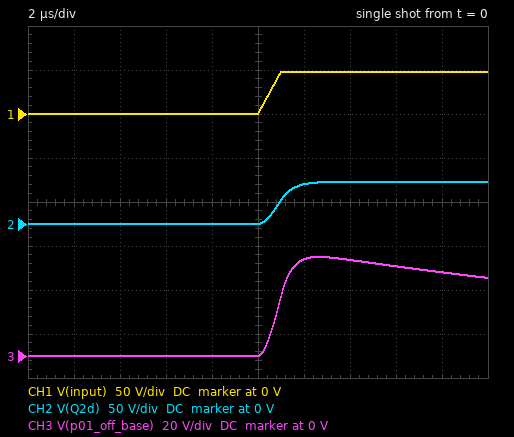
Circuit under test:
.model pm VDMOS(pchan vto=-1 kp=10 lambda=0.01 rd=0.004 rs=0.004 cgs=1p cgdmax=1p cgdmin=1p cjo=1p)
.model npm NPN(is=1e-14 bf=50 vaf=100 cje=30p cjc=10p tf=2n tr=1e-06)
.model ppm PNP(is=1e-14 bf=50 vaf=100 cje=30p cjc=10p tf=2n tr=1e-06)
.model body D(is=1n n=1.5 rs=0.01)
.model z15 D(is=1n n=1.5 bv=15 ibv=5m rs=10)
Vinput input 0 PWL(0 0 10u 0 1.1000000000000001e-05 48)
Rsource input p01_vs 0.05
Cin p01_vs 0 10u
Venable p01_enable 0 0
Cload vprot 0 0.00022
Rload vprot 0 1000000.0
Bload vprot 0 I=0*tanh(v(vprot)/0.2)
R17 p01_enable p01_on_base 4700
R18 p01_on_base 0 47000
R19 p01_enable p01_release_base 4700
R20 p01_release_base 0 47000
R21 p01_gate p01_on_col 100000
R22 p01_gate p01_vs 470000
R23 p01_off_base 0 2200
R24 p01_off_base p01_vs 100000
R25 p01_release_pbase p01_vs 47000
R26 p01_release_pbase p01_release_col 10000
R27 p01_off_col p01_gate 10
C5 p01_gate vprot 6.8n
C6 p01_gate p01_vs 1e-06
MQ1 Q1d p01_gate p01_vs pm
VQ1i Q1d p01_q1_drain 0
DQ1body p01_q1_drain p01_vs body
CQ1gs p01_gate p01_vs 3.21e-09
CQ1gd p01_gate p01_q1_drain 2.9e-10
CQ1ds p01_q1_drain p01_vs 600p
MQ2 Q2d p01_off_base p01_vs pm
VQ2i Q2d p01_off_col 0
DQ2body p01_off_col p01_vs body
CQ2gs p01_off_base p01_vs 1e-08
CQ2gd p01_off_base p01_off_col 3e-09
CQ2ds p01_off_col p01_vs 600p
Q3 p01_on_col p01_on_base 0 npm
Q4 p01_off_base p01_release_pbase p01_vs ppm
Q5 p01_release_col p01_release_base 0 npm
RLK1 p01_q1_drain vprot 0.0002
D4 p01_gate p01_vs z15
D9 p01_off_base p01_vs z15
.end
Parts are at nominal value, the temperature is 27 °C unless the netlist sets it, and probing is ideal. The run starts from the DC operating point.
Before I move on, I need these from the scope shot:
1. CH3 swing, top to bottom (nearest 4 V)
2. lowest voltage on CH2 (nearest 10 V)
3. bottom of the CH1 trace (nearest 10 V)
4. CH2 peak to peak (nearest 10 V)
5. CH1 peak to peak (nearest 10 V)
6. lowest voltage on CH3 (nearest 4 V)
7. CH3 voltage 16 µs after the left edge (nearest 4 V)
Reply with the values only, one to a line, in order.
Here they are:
44 V
0 V
0 V
50 V
50 V
0 V
40 V
